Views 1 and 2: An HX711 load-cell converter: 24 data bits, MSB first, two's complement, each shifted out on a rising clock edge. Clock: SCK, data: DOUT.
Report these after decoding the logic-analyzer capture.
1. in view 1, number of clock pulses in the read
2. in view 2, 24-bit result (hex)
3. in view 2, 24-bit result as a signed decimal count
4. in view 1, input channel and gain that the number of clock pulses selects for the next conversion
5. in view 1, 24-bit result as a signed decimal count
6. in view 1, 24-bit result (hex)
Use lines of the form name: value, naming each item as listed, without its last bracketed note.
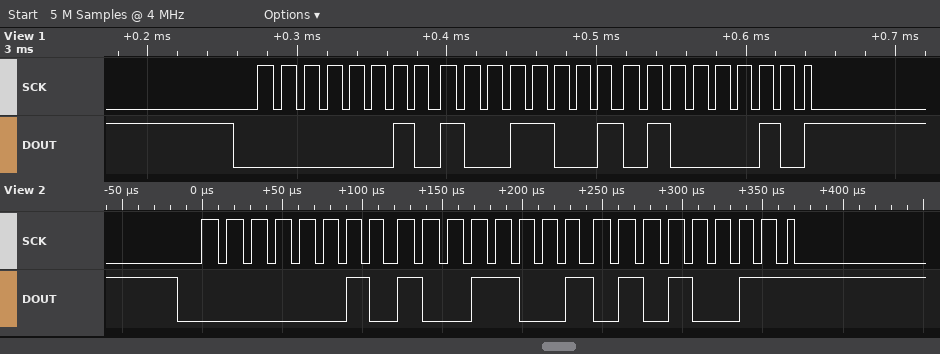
in view 1, number of clock pulses in the read: 25
in view 2, 24-bit result: 0x029953
in view 2, 24-bit result as a signed decimal count: 170323
in view 1, input channel and gain that the number of clock pulses selects for the next conversion: channel A, gain 128
in view 1, 24-bit result as a signed decimal count: 170306
in view 1, 24-bit result: 0x029942
